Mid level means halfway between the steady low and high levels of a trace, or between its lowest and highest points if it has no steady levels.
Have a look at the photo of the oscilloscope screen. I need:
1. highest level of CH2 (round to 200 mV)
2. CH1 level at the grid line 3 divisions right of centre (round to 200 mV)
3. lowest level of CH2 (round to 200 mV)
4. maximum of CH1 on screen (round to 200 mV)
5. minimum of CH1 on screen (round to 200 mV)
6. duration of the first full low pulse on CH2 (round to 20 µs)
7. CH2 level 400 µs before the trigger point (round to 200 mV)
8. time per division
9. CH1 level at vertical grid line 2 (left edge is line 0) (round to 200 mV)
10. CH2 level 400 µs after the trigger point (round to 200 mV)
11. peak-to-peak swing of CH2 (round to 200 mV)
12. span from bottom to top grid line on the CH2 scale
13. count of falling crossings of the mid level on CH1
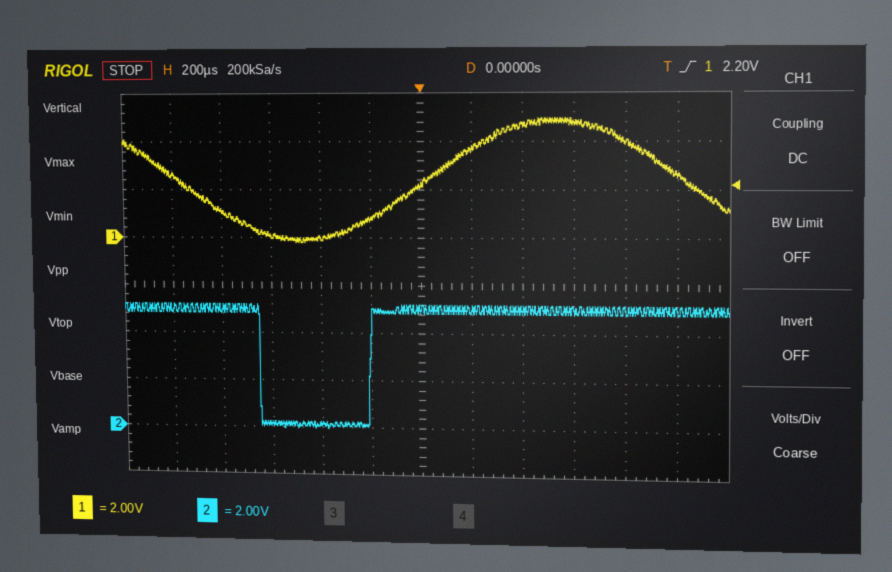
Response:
5.2 V
4.8 V
0.0 V
5.0 V
-200 mV
440 µs
200 mV
200 µs
1.2 V
5.0 V
5.2 V
16 V
2
